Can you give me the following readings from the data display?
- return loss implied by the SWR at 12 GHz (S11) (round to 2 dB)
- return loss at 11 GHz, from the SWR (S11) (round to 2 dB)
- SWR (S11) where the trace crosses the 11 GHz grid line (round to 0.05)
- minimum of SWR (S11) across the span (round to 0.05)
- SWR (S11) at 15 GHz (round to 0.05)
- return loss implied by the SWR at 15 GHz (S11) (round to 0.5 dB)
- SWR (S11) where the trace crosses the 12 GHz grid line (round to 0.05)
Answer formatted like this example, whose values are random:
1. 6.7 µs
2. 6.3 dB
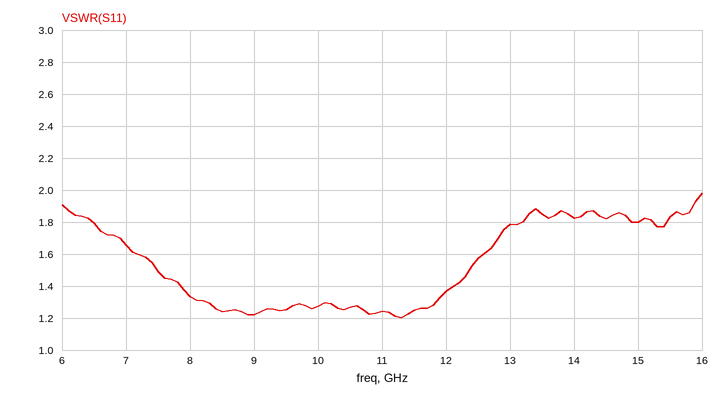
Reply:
1. 16 dB
2. 20 dB
3. 1.25
4. 1.20
5. 1.80
6. 11.0 dB
7. 1.35
